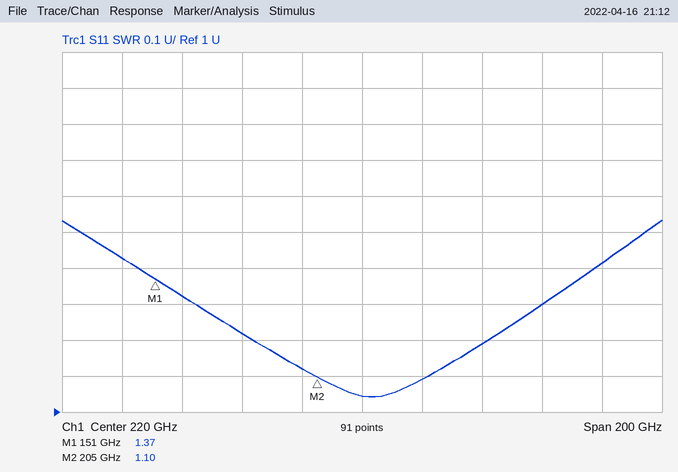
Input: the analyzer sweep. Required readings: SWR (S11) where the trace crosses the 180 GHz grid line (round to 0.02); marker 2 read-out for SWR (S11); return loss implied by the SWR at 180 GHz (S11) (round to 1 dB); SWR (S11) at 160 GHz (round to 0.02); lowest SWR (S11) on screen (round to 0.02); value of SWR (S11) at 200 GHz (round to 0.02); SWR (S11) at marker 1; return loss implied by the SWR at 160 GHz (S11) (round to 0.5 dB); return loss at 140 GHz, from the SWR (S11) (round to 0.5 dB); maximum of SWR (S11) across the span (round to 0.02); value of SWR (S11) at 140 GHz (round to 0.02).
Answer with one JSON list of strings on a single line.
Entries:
["1.22", "1.10", "20 dB", "1.32", "1.04", "1.12", "1.37", "17.0 dB", "15.0 dB", "1.54", "1.42"]
